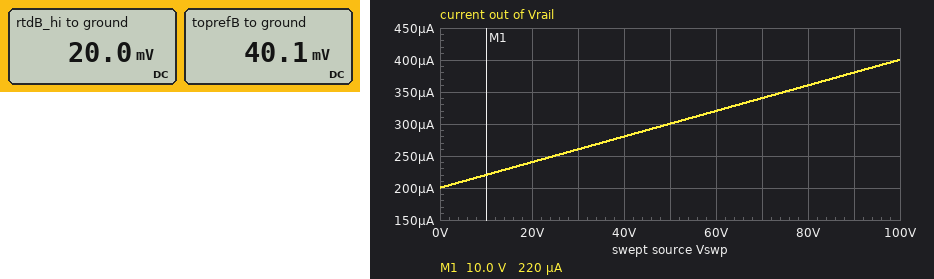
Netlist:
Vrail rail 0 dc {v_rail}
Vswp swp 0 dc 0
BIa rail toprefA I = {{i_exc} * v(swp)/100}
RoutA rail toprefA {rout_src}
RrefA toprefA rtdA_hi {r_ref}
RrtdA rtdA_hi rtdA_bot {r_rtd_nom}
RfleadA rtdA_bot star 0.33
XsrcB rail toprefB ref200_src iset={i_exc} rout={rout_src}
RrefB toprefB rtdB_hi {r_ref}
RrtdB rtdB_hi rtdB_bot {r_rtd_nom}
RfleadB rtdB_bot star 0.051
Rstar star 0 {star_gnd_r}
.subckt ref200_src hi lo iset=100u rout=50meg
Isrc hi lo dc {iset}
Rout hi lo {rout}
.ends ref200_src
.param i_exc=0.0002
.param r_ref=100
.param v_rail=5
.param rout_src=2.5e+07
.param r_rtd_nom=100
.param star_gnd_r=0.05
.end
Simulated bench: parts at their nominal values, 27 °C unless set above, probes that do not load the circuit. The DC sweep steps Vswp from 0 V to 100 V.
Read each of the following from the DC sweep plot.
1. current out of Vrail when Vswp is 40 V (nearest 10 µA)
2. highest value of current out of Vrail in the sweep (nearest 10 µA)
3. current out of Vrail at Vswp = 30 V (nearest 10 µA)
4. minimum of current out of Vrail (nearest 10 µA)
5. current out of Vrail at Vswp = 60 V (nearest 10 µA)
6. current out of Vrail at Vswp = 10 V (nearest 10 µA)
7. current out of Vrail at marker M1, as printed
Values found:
280 µA
400 µA
260 µA
200 µA
320 µA
220 µA
220 µA
